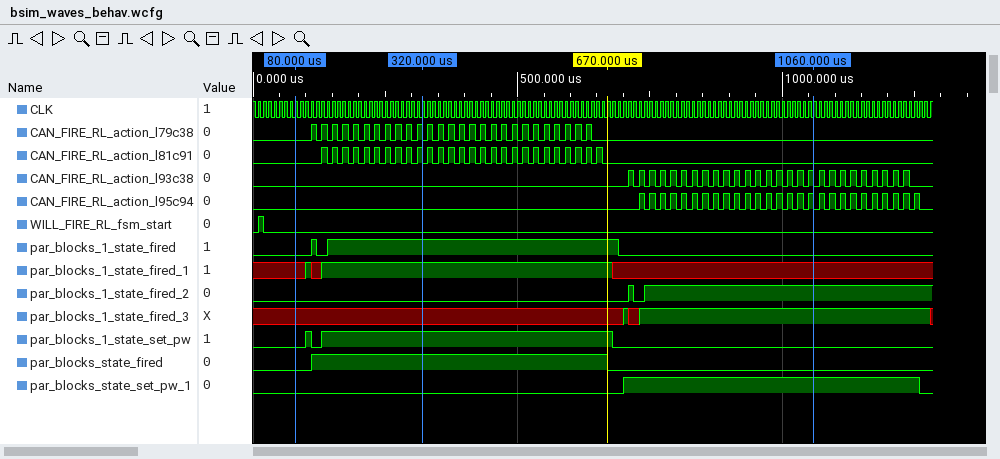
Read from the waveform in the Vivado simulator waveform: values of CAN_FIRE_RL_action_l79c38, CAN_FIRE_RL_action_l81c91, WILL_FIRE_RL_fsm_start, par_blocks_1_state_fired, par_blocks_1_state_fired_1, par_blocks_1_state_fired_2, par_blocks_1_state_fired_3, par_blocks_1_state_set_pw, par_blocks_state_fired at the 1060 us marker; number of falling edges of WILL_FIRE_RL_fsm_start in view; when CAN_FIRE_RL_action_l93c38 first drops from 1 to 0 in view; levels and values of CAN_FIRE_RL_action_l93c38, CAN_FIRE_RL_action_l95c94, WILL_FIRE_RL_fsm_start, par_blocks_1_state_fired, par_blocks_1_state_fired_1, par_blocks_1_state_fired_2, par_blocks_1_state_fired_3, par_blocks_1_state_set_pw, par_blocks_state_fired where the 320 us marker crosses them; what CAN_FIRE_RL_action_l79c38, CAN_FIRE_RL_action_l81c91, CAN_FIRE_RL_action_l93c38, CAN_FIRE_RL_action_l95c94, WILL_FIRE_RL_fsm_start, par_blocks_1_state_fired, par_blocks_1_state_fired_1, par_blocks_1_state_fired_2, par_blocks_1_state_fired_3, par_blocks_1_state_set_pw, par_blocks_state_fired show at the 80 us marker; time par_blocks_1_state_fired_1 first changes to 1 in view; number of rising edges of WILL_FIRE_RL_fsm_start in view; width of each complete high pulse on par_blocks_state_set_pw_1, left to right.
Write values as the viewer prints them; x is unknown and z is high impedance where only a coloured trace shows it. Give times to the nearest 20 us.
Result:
CAN_FIRE_RL_action_l79c38=0, CAN_FIRE_RL_action_l81c91=0, WILL_FIRE_RL_fsm_start=0, par_blocks_1_state_fired=0, par_blocks_1_state_fired_1=x, par_blocks_1_state_fired_2=1, par_blocks_1_state_fired_3=1, par_blocks_1_state_set_pw=0, par_blocks_state_fired=0
1
720 us
CAN_FIRE_RL_action_l93c38=0, CAN_FIRE_RL_action_l95c94=0, WILL_FIRE_RL_fsm_start=0, par_blocks_1_state_fired=1, par_blocks_1_state_fired_1=1, par_blocks_1_state_fired_2=0, par_blocks_1_state_fired_3=x, par_blocks_1_state_set_pw=1, par_blocks_state_fired=1
CAN_FIRE_RL_action_l79c38=0, CAN_FIRE_RL_action_l81c91=0, CAN_FIRE_RL_action_l93c38=0, CAN_FIRE_RL_action_l95c94=0, WILL_FIRE_RL_fsm_start=0, par_blocks_1_state_fired=0, par_blocks_1_state_fired_1=x, par_blocks_1_state_fired_2=0, par_blocks_1_state_fired_3=x, par_blocks_1_state_set_pw=0, par_blocks_state_fired=0
100 us
1
560 us
